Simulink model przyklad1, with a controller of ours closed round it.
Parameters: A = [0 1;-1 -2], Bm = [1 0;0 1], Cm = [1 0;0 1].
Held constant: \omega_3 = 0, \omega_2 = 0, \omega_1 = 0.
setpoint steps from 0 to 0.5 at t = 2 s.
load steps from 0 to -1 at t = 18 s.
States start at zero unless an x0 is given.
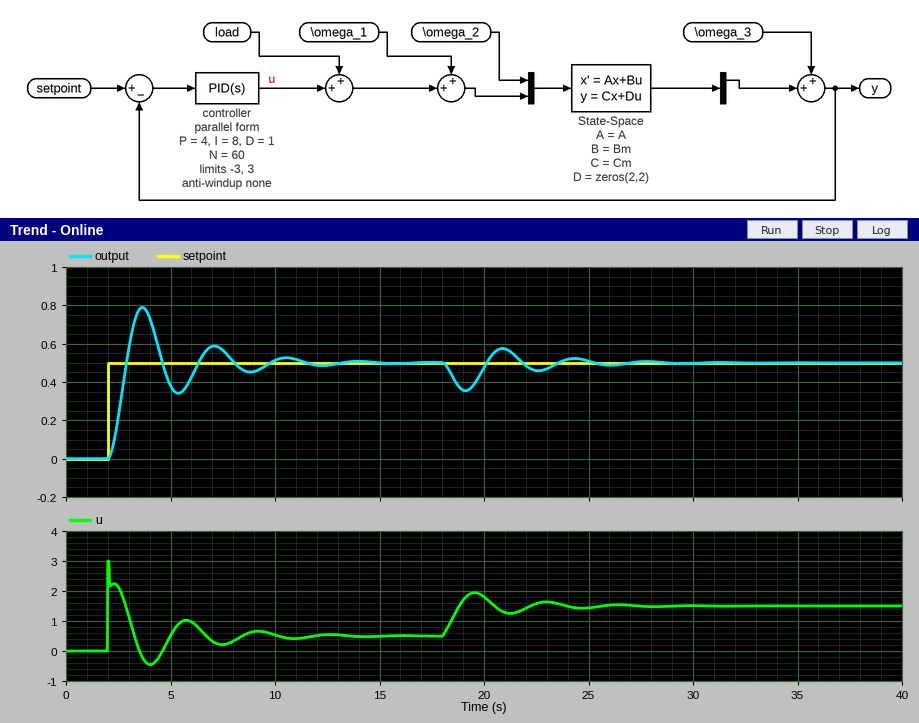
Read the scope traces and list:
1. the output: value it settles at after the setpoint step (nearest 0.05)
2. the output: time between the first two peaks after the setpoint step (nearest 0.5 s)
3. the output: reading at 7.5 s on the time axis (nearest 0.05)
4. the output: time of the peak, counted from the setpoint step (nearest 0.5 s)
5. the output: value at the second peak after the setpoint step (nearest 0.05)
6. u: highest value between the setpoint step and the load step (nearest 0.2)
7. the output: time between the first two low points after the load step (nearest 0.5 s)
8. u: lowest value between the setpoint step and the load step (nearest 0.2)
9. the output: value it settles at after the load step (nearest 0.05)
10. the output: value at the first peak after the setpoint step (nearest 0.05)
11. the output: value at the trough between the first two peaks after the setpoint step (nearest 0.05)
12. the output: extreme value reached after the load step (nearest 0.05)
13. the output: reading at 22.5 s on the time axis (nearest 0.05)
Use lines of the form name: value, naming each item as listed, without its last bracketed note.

the output: value it settles at after the setpoint step: 0.50
the output: time between the first two peaks after the setpoint step: 3.5 s
the output: reading at 7.5 s on the time axis: 0.55
the output: time of the peak, counted from the setpoint step: 1.5 s
the output: value at the second peak after the setpoint step: 0.60
u: highest value between the setpoint step and the load step: 3.0
the output: time between the first two low points after the load step: 3.5 s
u: lowest value between the setpoint step and the load step: -0.4
the output: value it settles at after the load step: 0.50
the output: value at the first peak after the setpoint step: 0.80
the output: value at the trough between the first two peaks after the setpoint step: 0.35
the output: extreme value reached after the load step: 0.35
the output: reading at 22.5 s on the time axis: 0.45
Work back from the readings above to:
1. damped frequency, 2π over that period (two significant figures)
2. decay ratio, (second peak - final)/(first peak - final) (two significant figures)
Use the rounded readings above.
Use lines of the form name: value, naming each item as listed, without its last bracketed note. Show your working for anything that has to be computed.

damped frequency, 2π over that period: 2π / 3.5 = 1.8 rad/s
decay ratio, (second peak - final)/(first peak - final): (0.6 - 0.5) / (0.8 - 0.5) = 0.33
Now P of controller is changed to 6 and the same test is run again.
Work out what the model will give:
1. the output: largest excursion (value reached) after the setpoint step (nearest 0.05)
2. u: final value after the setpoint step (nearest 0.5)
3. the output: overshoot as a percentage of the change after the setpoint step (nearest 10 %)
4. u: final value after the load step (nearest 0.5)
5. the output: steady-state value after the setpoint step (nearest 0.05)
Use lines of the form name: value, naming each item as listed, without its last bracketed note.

the output: largest excursion (value reached) after the setpoint step: 0.75
u: final value after the setpoint step: 0.5
the output: overshoot as a percentage of the change after the setpoint step: 50 %
u: final value after the load step: 1.5
the output: steady-state value after the setpoint step: 0.50
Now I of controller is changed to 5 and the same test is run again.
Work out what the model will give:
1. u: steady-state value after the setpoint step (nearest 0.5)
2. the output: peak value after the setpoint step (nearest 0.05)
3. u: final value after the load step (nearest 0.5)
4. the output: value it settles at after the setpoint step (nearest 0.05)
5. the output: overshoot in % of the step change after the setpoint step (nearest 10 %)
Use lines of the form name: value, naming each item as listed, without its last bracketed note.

u: steady-state value after the setpoint step: 0.5
the output: peak value after the setpoint step: 0.70
u: final value after the load step: 1.5
the output: value it settles at after the setpoint step: 0.50
the output: overshoot in % of the step change after the setpoint step: 40 %
